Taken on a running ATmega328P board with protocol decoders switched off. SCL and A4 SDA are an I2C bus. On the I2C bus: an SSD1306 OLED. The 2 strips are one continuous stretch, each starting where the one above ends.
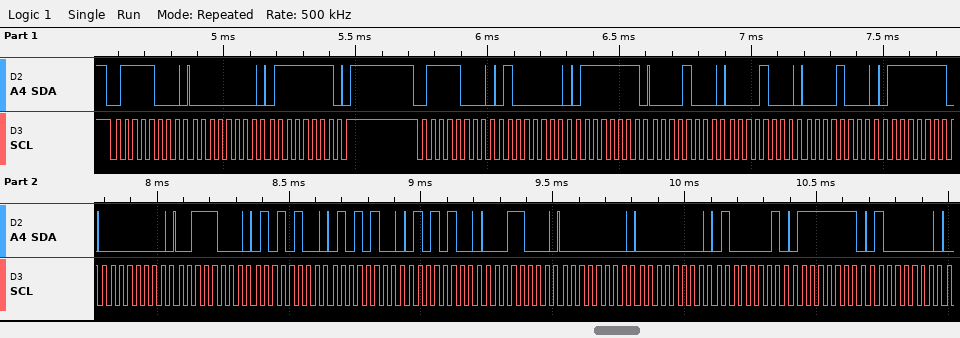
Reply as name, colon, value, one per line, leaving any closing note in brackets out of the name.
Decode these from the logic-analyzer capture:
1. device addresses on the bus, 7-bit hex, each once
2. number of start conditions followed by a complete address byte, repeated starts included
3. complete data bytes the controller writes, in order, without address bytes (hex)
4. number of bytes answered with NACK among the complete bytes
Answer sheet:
device addresses on the bus, 7-bit hex, each once: 0x3C
number of start conditions followed by a complete address byte, repeated starts included: 2
complete data bytes the controller writes, in order, without address bytes: 00 7F 40 7F 08 08 08 7F 00 38 54 54 54 18 00 00 41 7F 40
number of bytes answered with NACK among the complete bytes: 0
